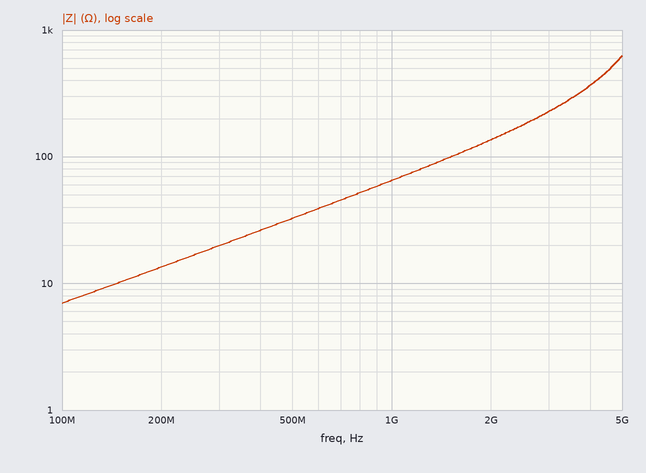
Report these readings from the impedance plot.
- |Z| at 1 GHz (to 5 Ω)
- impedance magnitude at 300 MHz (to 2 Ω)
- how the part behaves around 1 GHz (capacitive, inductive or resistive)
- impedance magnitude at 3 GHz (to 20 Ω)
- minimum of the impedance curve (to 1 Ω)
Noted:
65 Ω
20 Ω
inductive
220 Ω
7 Ω
